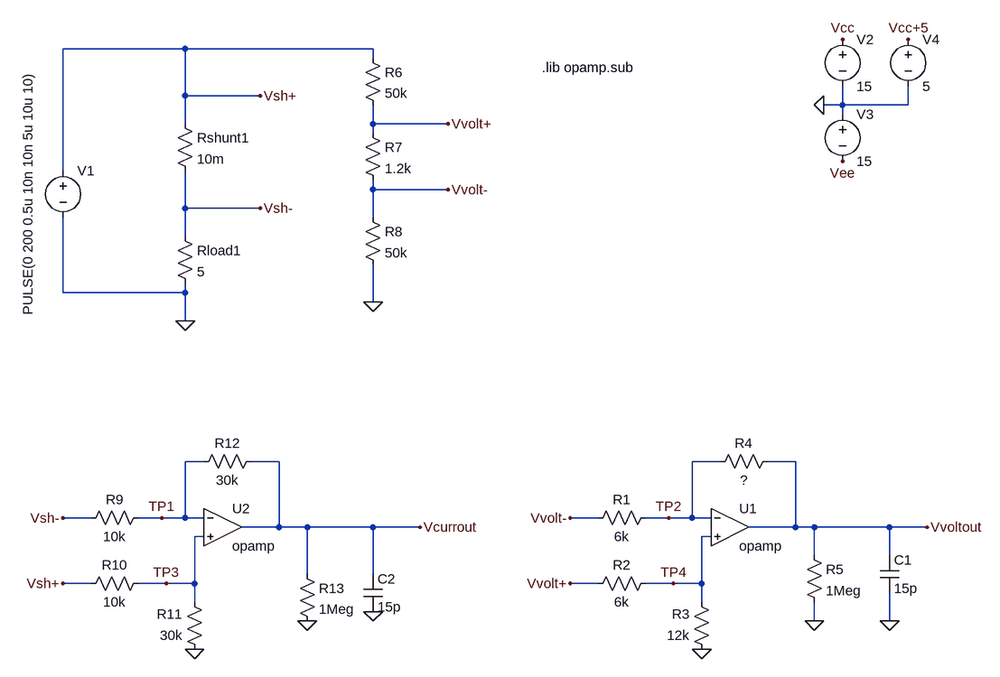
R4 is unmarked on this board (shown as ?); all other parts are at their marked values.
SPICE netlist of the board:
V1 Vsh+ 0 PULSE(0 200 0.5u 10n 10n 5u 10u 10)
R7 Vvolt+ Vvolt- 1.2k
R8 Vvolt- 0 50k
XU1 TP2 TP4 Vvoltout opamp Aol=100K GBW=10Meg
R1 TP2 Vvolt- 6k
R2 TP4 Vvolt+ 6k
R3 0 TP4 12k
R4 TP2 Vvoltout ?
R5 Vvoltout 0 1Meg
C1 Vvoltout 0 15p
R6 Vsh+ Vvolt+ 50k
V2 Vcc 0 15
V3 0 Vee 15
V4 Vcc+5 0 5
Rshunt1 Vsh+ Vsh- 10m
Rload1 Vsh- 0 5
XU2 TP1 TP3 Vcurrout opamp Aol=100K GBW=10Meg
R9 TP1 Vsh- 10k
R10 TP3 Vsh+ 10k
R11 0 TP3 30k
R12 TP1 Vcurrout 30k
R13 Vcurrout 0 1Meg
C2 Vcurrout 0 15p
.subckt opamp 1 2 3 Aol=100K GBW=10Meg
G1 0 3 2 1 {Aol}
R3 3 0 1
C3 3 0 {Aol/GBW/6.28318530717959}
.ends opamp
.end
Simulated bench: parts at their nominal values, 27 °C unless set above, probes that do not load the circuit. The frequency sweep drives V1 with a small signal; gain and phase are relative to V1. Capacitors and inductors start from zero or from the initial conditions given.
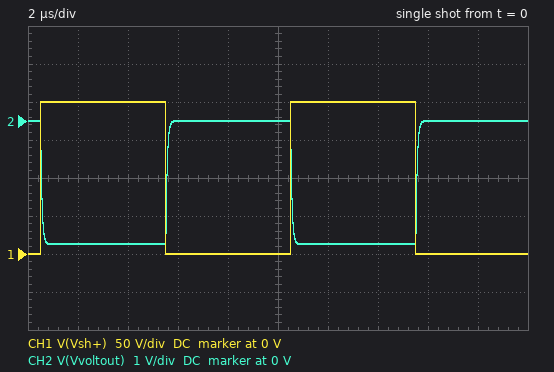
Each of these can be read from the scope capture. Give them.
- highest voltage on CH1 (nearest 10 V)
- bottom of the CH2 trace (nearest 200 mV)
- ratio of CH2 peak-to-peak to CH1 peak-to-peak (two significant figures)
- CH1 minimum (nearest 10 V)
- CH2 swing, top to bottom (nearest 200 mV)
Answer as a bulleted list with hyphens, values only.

- 200 V
- -3.2 V
- 0.016
- 0 V
- 3.2 V
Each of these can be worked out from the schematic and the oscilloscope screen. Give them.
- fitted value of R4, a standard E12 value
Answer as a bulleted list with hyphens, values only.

- 18 kΩ
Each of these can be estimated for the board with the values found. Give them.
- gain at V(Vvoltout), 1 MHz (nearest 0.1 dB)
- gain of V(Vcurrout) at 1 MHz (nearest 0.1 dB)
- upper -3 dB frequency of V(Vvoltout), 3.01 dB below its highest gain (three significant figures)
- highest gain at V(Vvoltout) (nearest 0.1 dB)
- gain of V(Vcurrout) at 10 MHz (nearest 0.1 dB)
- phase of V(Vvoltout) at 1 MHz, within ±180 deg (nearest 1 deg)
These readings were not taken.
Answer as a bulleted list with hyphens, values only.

- -36.3 dB
- -45.1 dB
- 2.94 MHz
- -35.8 dB
- -56.8 dB
- 161 deg
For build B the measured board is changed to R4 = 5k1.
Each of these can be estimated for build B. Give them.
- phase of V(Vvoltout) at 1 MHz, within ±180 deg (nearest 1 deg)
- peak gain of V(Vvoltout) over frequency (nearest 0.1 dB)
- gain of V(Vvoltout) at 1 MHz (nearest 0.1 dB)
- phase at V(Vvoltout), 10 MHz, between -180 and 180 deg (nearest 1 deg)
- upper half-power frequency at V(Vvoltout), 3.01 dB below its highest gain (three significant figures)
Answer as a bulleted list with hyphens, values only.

- -12 deg
- -23.7 dB
- -23.9 dB
- -65 deg
- 4.64 MHz
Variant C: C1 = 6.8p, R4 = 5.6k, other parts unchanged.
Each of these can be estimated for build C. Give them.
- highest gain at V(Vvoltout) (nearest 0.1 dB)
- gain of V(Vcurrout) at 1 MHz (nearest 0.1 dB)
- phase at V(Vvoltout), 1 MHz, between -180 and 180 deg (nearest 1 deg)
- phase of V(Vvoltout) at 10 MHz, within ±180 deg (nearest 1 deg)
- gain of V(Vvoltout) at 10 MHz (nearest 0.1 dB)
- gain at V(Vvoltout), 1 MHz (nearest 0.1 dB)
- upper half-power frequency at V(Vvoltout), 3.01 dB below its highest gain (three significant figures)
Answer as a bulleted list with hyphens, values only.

- -24.2 dB
- -45.1 dB
- -12 deg
- -66 deg
- -31.8 dB
- -24.4 dB
- 4.54 MHz
